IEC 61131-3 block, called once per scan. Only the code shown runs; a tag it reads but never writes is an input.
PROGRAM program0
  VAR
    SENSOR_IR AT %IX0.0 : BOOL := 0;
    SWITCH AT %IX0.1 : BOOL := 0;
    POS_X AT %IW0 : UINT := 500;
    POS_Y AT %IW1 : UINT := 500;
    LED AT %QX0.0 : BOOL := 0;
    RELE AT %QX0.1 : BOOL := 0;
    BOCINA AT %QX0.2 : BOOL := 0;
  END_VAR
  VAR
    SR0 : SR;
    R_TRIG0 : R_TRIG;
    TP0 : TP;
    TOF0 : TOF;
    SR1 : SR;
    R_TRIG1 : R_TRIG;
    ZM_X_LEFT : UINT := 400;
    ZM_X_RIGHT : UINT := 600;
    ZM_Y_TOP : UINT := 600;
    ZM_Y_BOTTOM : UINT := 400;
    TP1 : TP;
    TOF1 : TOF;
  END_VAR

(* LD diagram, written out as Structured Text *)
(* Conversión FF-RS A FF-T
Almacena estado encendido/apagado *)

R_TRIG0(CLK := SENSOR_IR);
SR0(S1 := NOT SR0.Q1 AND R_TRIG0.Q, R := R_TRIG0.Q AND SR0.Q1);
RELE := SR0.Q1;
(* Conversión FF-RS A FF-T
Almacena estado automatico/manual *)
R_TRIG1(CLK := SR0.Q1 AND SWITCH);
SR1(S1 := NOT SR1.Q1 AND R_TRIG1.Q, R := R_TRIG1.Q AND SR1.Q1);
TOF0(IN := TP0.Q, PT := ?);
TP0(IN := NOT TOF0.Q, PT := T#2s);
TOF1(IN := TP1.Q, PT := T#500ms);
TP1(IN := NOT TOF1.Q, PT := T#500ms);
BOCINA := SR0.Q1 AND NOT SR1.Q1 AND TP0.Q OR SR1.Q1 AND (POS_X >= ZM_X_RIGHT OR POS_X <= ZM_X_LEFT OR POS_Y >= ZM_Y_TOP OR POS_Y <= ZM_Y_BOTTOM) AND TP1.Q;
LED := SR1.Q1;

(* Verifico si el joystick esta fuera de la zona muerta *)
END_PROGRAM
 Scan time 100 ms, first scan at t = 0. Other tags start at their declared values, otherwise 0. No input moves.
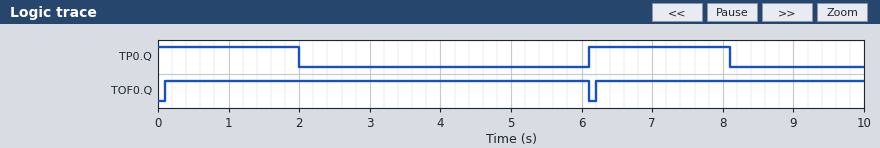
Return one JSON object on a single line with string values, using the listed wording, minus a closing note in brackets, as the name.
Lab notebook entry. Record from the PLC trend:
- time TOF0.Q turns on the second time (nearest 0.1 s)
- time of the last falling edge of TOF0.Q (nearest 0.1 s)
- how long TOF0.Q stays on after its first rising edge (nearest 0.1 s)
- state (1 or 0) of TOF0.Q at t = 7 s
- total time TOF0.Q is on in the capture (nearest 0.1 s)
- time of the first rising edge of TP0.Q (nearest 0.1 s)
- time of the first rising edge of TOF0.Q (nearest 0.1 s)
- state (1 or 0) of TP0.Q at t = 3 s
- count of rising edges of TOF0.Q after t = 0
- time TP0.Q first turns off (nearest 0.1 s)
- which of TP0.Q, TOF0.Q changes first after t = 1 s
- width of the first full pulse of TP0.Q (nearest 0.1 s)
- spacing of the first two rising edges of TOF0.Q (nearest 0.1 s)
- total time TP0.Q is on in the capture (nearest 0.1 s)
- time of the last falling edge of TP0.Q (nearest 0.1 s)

{"time TOF0.Q turns on the second time": "6.2 s", "time of the last falling edge of TOF0.Q": "6.1 s", "how long TOF0.Q stays on after its first rising edge": "6.0 s", "state (1 or 0) of TOF0.Q at t = 7 s": "1", "total time TOF0.Q is on in the capture": "9.8 s", "time of the first rising edge of TP0.Q": "6.1 s", "time of the first rising edge of TOF0.Q": "0.1 s", "state (1 or 0) of TP0.Q at t = 3 s": "0", "count of rising edges of TOF0.Q after t = 0": "2", "time TP0.Q first turns off": "2.0 s", "which of TP0.Q, TOF0.Q changes first after t = 1 s": "TP0.Q", "width of the first full pulse of TP0.Q": "2.0 s", "spacing of the first two rising edges of TOF0.Q": "6.1 s", "total time TP0.Q is on in the capture": "4.0 s", "time of the last falling edge of TP0.Q": "8.1 s"}
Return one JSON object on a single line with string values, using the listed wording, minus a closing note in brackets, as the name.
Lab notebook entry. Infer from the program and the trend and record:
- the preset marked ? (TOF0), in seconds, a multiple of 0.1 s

{"the preset marked ? (TOF0), in seconds, a multiple of 0.1 s": "4.0 s"}
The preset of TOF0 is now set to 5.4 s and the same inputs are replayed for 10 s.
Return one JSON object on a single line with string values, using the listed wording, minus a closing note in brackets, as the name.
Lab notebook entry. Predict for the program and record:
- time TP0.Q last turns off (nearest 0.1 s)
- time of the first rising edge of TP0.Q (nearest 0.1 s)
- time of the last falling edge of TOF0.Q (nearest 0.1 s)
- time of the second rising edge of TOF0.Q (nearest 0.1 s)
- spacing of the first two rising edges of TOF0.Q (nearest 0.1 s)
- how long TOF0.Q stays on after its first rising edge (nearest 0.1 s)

{"time TP0.Q last turns off": "9.5 s", "time of the first rising edge of TP0.Q": "7.5 s", "time of the last falling edge of TOF0.Q": "7.5 s", "time of the second rising edge of TOF0.Q": "7.6 s", "spacing of the first two rising edges of TOF0.Q": "7.5 s", "how long TOF0.Q stays on after its first rising edge": "7.4 s"}
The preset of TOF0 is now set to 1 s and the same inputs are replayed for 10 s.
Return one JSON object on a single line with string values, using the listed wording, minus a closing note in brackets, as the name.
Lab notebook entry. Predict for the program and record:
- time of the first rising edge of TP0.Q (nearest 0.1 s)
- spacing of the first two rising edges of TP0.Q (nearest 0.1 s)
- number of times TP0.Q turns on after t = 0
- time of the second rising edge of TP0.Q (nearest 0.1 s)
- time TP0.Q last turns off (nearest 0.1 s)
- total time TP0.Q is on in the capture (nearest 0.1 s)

{"time of the first rising edge of TP0.Q": "3.1 s", "spacing of the first two rising edges of TP0.Q": "3.1 s", "number of times TP0.Q turns on after t = 0": "3", "time of the second rising edge of TP0.Q": "6.2 s", "time TP0.Q last turns off": "8.2 s", "total time TP0.Q is on in the capture": "6.7 s"}
